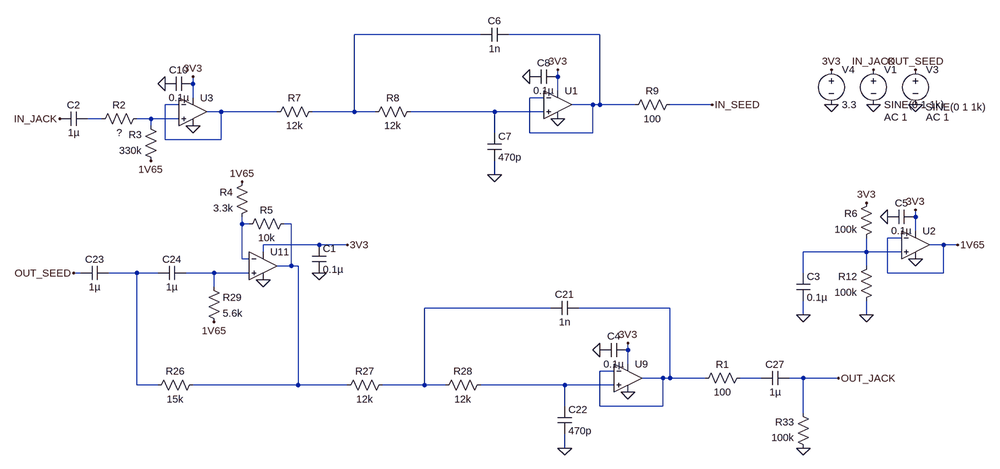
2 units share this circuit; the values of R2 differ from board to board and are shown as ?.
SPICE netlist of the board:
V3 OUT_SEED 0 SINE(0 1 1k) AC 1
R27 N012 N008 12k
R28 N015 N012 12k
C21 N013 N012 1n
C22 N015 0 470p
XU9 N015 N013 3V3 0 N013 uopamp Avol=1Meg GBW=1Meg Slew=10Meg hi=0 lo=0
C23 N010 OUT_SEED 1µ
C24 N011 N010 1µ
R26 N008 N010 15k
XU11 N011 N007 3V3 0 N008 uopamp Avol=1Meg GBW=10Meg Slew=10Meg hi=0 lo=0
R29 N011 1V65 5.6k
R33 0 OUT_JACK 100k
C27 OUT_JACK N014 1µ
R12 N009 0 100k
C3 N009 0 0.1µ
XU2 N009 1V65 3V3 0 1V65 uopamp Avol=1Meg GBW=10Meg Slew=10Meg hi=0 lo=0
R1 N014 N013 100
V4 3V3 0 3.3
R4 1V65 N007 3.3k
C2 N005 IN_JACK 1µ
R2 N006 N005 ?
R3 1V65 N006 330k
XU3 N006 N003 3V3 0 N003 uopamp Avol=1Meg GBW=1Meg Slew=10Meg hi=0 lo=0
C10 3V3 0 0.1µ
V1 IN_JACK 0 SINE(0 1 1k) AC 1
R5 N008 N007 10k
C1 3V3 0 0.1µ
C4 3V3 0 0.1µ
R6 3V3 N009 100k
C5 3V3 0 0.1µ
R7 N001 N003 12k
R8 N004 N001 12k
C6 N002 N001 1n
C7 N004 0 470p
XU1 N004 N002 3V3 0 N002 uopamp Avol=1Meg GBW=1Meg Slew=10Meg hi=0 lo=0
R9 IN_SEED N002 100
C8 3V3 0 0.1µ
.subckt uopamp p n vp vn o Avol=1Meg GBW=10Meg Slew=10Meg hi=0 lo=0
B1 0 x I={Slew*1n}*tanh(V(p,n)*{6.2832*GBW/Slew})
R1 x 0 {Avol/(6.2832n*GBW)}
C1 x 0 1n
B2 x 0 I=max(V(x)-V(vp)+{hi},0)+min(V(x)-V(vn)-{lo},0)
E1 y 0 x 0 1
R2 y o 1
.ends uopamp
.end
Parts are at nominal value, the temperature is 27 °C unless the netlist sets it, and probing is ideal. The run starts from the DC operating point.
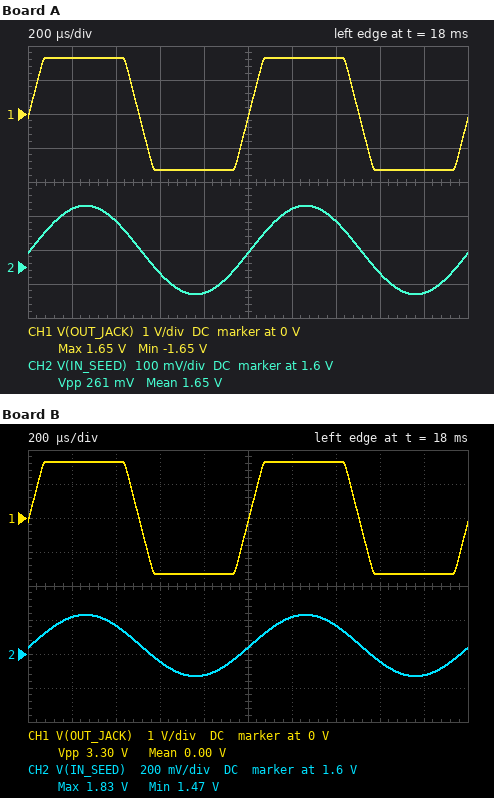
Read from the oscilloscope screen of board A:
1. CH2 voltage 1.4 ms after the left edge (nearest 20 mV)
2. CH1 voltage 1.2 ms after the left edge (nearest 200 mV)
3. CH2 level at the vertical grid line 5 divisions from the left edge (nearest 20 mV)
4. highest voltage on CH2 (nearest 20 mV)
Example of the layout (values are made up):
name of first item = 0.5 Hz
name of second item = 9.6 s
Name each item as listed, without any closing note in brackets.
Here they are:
CH2 voltage 1.4 ms after the left edge = 1.74 V
CH1 voltage 1.2 ms after the left edge = 1.6 V
CH2 level at the vertical grid line 5 divisions from the left edge = 1.64 V
highest voltage on CH2 = 1.78 V
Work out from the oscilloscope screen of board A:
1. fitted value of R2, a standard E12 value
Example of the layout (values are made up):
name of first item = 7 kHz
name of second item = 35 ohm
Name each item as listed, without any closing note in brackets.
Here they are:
fitted value of R2, a standard E12 value = 2.2 MΩ
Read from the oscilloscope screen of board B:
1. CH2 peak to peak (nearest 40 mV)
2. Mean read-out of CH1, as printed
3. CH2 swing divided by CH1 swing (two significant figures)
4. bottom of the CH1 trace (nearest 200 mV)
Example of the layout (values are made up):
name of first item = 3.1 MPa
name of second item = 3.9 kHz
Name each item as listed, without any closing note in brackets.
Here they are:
CH2 peak to peak = 360 mV
Mean read-out of CH1, as printed = 0.00 V
CH2 swing divided by CH1 swing = 0.11
bottom of the CH1 trace = -1.6 V
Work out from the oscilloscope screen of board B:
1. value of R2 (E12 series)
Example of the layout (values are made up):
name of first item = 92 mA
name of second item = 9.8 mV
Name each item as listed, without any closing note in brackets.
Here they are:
value of R2 = 1.5 MΩ
